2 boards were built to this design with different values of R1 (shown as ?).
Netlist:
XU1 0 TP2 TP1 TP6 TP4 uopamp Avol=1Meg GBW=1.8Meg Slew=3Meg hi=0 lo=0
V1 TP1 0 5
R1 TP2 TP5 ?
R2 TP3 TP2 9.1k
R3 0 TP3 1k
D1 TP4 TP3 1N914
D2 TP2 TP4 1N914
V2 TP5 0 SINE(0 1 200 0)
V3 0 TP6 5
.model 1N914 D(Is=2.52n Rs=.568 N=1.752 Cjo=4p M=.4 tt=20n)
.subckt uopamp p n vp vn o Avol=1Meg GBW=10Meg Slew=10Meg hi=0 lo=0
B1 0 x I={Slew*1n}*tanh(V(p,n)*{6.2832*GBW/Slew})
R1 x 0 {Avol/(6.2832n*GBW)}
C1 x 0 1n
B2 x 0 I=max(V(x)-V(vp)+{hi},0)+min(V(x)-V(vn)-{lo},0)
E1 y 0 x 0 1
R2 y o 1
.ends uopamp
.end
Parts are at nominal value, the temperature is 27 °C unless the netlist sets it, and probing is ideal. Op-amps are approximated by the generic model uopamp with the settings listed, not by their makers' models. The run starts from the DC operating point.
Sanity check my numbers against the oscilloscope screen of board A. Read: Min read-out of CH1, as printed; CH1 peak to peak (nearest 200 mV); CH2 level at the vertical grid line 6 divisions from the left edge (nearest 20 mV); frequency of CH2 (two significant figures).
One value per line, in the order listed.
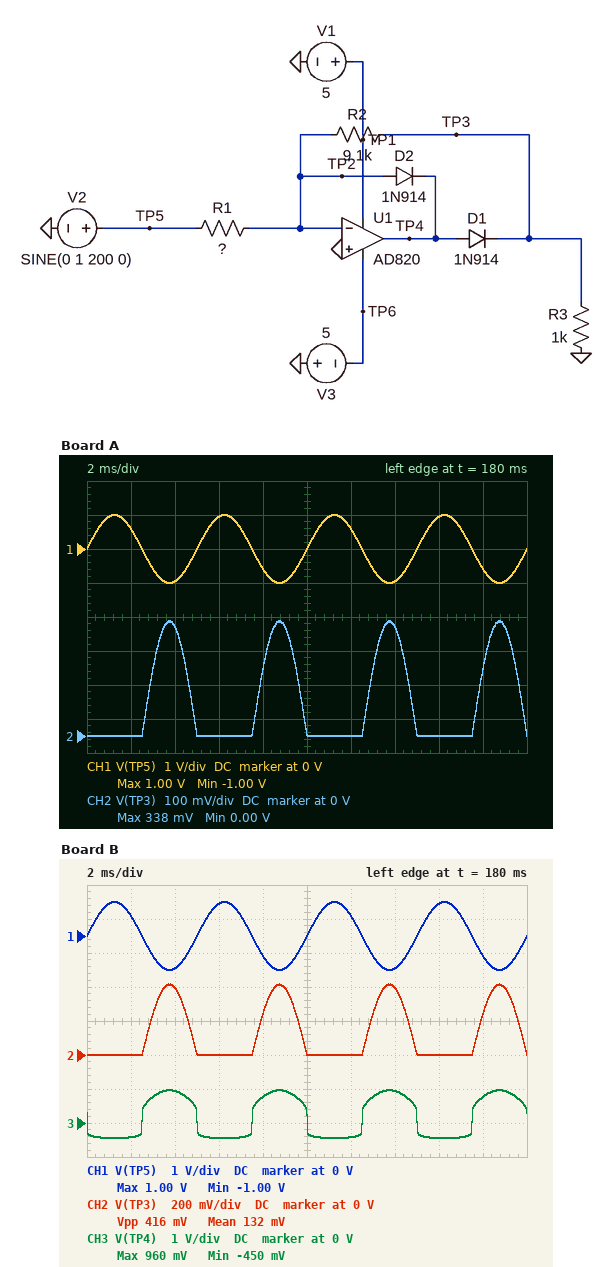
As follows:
-1.00 V
2.0 V
0 V
200 Hz
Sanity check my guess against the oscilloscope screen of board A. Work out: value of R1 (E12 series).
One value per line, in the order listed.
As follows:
27 kΩ
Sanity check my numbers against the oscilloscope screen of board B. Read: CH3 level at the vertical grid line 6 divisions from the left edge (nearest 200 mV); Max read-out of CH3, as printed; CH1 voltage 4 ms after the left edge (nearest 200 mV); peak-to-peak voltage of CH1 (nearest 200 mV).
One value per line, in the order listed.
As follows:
-400 mV
960 mV
-1.0 V
2.0 V
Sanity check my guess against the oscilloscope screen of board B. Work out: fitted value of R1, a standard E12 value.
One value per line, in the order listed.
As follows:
22 kΩ
